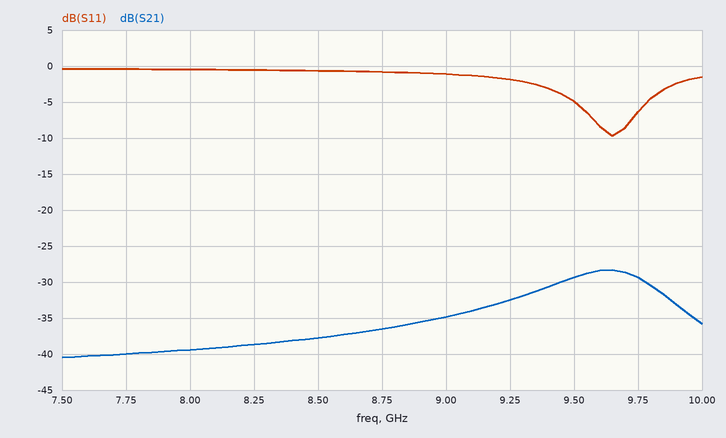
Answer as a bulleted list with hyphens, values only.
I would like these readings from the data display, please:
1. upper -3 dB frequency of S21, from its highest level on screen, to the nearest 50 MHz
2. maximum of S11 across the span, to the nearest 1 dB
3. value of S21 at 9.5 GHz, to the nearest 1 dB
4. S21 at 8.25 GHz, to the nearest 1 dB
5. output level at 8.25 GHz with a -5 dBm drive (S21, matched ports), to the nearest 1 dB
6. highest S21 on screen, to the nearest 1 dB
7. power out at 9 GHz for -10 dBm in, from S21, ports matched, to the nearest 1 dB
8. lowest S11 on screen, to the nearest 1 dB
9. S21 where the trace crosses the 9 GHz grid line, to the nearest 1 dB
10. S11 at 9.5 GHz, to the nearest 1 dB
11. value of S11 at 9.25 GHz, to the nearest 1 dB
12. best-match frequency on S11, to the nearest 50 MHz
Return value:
- 9.85 GHz
- 0 dB
- -29 dB
- -39 dB
- -44 dBm
- -28 dB
- -45 dBm
- -10 dB
- -35 dB
- -5 dB
- -2 dB
- 9.65 GHz
